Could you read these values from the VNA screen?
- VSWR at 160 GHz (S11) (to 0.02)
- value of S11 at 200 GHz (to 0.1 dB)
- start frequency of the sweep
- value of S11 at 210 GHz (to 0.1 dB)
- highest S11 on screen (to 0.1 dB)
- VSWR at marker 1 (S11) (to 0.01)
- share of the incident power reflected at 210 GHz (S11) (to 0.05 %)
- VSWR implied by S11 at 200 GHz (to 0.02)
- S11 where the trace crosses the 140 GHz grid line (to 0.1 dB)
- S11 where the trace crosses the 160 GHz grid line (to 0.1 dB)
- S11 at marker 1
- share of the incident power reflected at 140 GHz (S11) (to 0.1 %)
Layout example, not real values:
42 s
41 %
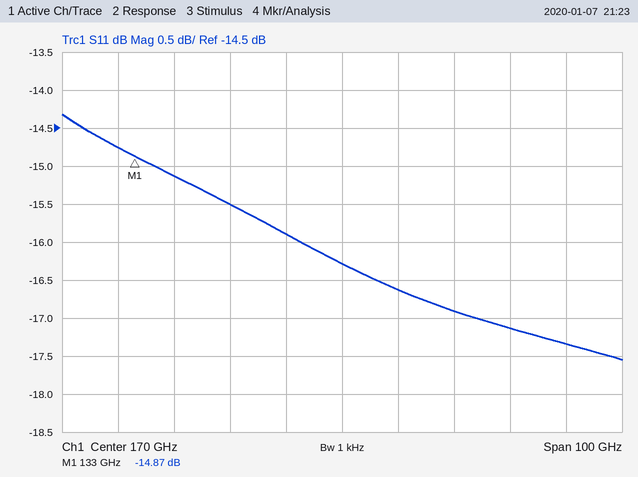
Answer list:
1.38
-17.1 dB
120 GHz
-17.3 dB
-14.3 dB
1.44
1.85 %
1.32
-15.1 dB
-15.9 dB
-14.87 dB
3.1 %
